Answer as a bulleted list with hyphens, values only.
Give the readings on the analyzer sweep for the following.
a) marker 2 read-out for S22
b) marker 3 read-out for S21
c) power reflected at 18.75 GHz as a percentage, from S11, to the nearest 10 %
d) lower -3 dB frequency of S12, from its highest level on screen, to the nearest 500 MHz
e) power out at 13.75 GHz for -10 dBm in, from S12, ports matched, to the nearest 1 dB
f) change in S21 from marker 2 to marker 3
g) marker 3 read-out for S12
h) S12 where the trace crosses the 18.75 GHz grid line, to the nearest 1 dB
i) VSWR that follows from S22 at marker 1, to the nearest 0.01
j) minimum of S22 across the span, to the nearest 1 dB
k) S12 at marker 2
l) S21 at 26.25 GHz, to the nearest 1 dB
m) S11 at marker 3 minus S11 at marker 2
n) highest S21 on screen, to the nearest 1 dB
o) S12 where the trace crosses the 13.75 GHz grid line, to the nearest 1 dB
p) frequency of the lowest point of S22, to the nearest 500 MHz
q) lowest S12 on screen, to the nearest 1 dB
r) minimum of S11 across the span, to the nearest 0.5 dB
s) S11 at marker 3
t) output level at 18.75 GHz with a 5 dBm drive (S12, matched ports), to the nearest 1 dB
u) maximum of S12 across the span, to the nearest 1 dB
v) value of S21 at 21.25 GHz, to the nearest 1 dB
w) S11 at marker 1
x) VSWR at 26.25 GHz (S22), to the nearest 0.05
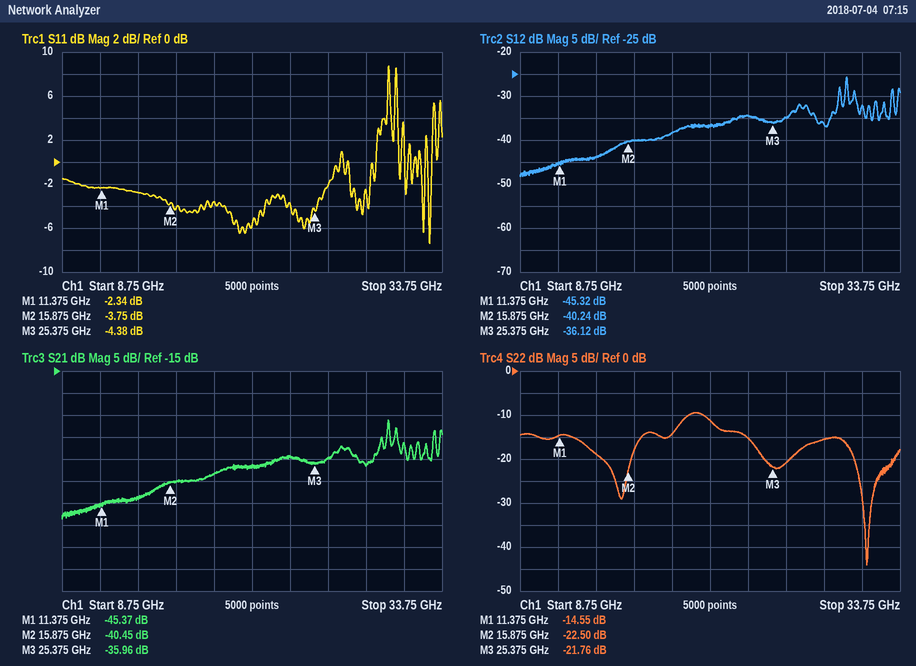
- -22.50 dB
- -35.96 dB
- 40 %
- 30.0 GHz
- -54 dBm
- 4.49 dB
- -36.12 dB
- -38 dB
- 1.46
- -44 dB
- -40.24 dB
- -35 dB
- -0.63 dB
- -26 dB
- -44 dB
- 31.5 GHz
- -48 dB
- -7.5 dB
- -4.38 dB
- -33 dBm
- -26 dB
- -37 dB
- -2.34 dB
- 1.20
